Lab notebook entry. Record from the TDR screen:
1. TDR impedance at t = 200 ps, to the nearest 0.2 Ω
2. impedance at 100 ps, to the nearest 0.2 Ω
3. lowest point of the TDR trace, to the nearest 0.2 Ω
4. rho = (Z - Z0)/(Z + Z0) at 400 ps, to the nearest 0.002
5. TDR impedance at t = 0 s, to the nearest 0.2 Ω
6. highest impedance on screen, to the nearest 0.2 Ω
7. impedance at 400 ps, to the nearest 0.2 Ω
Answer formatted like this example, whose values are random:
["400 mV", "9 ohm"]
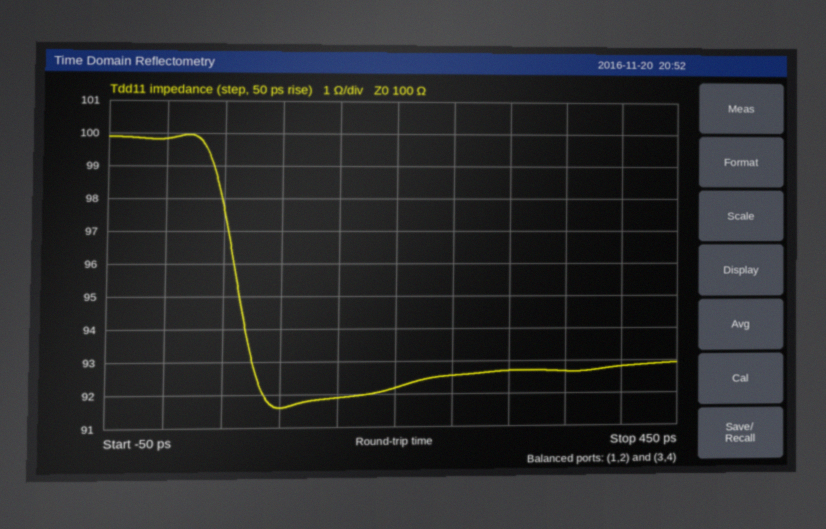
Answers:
["92.2 Ω", "91.6 Ω", "91.6 Ω", "-0.038", "99.8 Ω", "100.0 Ω", "92.8 Ω"]
